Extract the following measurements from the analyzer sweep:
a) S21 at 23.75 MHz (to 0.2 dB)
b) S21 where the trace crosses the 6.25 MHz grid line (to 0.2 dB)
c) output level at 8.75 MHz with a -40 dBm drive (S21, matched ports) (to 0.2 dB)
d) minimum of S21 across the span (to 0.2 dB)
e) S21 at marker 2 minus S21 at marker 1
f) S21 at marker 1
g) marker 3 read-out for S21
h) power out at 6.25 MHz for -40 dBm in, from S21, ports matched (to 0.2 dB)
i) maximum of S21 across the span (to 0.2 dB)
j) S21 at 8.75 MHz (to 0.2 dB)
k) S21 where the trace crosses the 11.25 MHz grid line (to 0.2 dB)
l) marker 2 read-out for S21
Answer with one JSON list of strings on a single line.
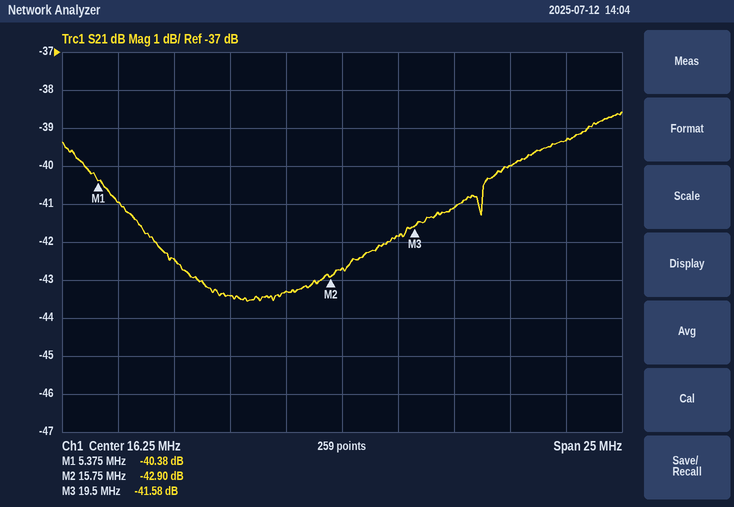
["-40.0 dB", "-41.0 dB", "-82.4 dBm", "-43.6 dB", "-2.52 dB", "-40.38 dB", "-41.58 dB", "-81.0 dBm", "-38.6 dB", "-42.4 dB", "-43.4 dB", "-42.90 dB"]
